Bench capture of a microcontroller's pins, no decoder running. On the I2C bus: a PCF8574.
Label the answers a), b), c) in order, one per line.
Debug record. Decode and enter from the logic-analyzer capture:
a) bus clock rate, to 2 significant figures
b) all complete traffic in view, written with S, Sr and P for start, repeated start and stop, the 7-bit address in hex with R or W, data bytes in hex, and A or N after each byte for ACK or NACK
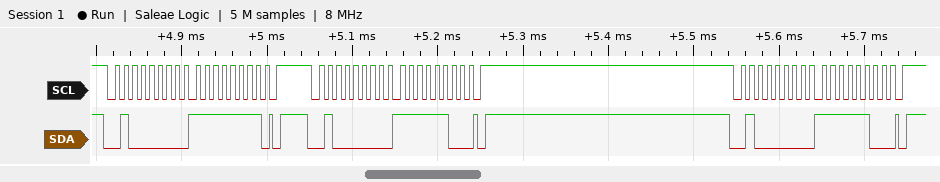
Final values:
a) 100 kHz
b) S 20W A FF A P S 20W A FC A P S 20W A FC A P
